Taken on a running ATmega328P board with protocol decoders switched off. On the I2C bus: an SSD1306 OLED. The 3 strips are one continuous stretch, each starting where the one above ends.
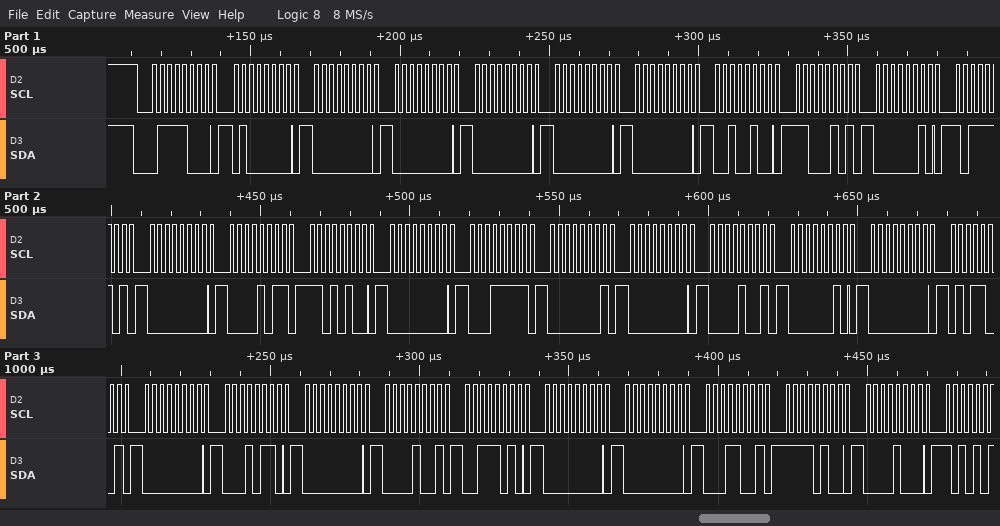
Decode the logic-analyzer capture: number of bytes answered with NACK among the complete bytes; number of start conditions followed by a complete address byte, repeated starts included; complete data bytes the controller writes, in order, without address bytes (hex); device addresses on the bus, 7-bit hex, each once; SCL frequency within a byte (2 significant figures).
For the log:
0
1
40 00 00 00 00 00 24 C5 02 BD 00 0B D4 00 1F 01 00 09 02 00 59 00 16 00 09 3A 00 00 19 F4 08
0x3C
400 kHz
